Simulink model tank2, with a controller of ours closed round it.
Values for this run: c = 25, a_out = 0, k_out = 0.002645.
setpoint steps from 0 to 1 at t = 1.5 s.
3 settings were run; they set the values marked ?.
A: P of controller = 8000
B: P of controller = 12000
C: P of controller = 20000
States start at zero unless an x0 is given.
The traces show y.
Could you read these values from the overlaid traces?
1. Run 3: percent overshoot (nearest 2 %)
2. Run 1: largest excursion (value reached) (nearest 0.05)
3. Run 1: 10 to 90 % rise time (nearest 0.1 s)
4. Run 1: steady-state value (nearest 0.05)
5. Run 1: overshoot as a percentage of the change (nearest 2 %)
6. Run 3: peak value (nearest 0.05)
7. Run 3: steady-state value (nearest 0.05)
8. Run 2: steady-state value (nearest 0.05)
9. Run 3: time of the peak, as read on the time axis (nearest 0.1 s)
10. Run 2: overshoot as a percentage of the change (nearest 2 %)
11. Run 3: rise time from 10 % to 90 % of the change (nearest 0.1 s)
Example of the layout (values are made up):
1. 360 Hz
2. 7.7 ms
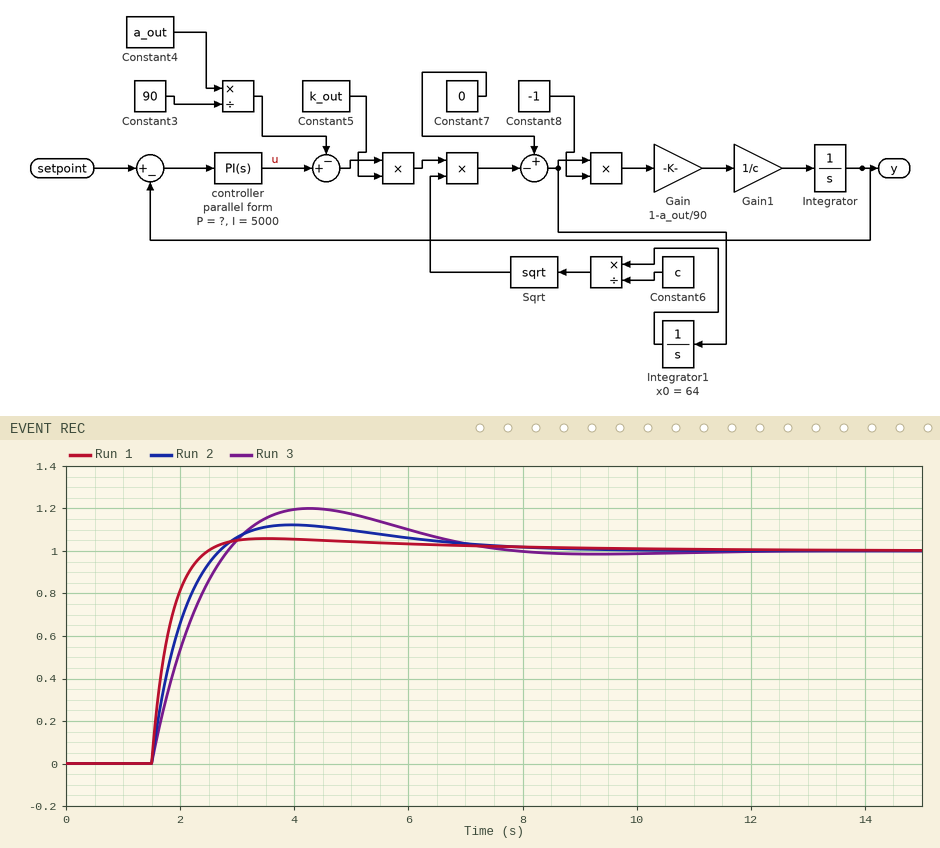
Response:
1. 20 %
2. 1.05
3. 0.6 s
4. 1.00
5. 6 %
6. 1.20
7. 1.00
8. 1.00
9. 4.3 s
10. 12 %
11. 1.0 s
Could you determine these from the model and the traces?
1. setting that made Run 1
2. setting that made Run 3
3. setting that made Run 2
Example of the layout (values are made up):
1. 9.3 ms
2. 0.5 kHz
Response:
1. C
2. A
3. B
